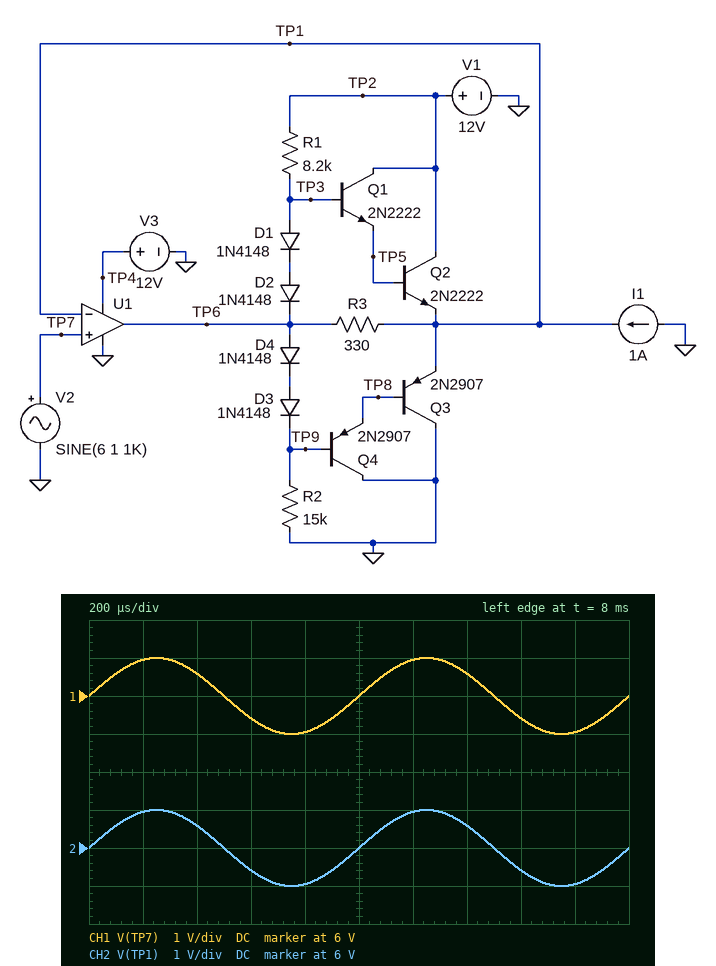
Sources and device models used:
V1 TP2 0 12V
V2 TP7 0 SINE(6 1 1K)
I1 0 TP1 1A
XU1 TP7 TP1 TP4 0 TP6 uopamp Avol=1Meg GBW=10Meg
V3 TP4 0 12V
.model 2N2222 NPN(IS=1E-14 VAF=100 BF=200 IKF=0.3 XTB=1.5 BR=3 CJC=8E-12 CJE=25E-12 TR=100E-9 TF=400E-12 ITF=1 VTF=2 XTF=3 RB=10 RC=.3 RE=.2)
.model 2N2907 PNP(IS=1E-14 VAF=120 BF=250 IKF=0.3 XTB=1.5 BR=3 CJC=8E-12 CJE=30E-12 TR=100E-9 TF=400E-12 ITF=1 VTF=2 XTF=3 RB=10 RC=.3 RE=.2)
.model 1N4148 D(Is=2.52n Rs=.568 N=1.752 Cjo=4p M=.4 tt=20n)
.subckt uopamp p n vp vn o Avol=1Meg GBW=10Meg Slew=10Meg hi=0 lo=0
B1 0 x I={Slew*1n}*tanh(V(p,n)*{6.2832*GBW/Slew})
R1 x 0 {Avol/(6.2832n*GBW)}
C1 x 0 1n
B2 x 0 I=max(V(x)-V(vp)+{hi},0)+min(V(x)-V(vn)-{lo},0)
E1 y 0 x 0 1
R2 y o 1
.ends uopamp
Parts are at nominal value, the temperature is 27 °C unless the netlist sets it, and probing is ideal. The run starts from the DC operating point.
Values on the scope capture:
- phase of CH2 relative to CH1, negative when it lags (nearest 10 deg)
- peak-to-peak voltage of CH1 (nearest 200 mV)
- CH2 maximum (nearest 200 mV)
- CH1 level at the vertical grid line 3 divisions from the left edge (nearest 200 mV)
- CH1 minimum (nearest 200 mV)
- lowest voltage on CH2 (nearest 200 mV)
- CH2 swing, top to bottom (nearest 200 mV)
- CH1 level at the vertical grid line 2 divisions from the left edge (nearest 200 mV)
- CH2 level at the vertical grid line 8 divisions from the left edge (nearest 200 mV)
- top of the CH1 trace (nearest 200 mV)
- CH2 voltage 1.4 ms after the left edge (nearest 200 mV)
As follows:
0 deg
2.0 V
7.0 V
5.4 V
5.0 V
5.0 V
2.0 V
6.6 V
5.4 V
7.0 V
6.6 V
